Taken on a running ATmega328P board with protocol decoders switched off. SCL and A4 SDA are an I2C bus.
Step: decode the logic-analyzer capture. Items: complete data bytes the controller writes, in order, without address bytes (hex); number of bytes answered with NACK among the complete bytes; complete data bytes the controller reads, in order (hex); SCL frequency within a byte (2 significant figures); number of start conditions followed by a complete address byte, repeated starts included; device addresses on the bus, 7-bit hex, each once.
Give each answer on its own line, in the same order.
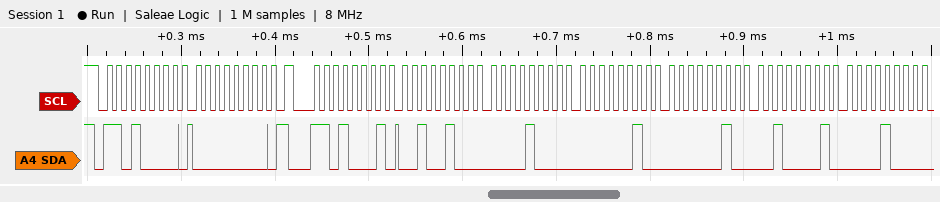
00
0
24 08 02 02 21 08
100 kHz
2
0x68
